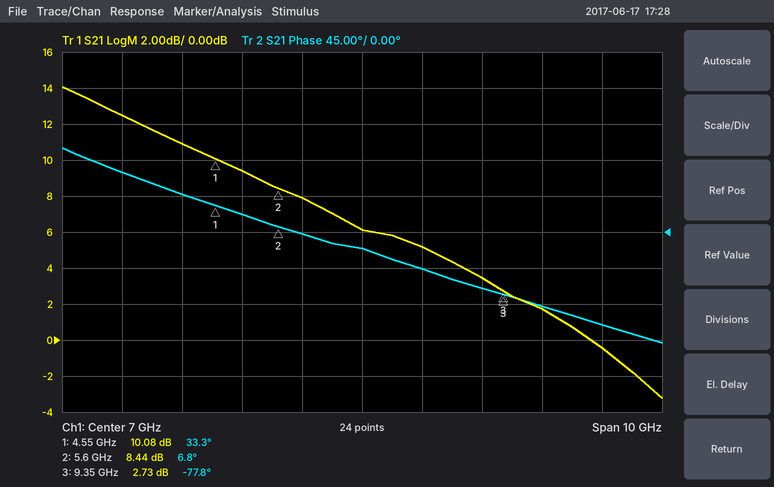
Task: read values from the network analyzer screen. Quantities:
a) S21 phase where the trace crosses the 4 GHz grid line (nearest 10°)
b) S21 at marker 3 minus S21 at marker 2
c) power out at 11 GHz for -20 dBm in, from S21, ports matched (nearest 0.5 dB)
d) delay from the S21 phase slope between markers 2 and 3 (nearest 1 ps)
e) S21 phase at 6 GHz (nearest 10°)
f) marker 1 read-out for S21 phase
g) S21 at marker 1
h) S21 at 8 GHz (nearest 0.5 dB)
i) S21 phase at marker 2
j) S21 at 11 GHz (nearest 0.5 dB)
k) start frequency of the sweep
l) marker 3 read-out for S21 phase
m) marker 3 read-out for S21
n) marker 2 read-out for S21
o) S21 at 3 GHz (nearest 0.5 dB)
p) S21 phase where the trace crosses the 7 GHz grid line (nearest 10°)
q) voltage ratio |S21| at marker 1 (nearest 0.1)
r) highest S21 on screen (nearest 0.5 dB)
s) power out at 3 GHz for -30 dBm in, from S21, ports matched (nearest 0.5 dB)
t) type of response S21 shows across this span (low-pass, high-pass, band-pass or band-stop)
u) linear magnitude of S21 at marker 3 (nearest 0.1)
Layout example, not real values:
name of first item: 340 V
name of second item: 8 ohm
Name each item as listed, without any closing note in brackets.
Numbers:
S21 phase where the trace crosses the 4 GHz grid line: 50°
S21 at marker 3 minus S21 at marker 2: -5.71 dB
power out at 11 GHz for -20 dBm in, from S21, ports matched: -20.5 dBm
delay from the S21 phase slope between markers 2 and 3: 63 ps
S21 phase at 6 GHz: 0°
marker 1 read-out for S21 phase: 33.3°
S21 at marker 1: 10.08 dB
S21 at 8 GHz: 5.0 dB
S21 phase at marker 2: 6.8°
S21 at 11 GHz: -0.5 dB
start frequency of the sweep: 2 GHz
marker 3 read-out for S21 phase: -77.8°
marker 3 read-out for S21: 2.73 dB
marker 2 read-out for S21: 8.44 dB
S21 at 3 GHz: 12.5 dB
S21 phase where the trace crosses the 7 GHz grid line: -20°
voltage ratio |S21| at marker 1: 3.2
highest S21 on screen: 14.0 dB
power out at 3 GHz for -30 dBm in, from S21, ports matched: -17.5 dBm
type of response S21 shows across this span: low-pass
linear magnitude of S21 at marker 3: 1.4
